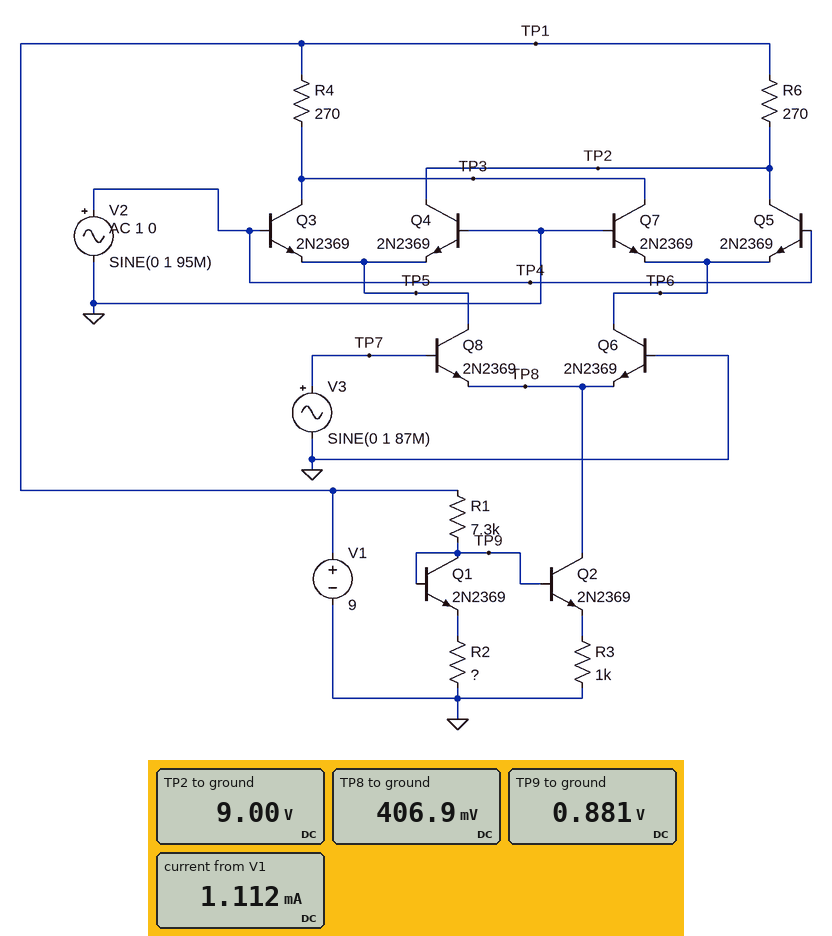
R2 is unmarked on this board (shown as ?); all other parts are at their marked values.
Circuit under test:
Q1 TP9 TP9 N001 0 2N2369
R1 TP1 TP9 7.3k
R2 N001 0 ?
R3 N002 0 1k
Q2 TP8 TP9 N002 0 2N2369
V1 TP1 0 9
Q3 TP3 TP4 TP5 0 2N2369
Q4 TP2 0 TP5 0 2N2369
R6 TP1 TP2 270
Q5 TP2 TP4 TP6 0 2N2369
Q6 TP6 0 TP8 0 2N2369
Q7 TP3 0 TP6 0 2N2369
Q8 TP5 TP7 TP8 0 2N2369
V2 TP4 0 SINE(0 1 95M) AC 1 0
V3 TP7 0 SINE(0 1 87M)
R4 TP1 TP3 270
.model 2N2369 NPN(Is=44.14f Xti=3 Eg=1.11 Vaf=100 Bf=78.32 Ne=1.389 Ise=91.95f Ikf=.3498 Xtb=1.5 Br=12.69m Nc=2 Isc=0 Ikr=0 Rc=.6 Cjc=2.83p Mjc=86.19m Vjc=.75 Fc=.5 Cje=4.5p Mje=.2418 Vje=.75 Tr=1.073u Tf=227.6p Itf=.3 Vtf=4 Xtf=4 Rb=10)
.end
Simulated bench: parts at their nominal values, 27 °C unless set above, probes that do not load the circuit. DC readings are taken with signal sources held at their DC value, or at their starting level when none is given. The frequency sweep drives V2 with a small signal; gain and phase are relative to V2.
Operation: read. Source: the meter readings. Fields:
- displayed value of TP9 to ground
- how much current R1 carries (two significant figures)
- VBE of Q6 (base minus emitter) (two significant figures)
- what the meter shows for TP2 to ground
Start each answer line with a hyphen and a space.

- 0.881 V
- 1.1 mA
- -410 mV
- 9.00 V
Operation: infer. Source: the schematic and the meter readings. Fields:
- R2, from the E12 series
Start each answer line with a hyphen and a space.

- 330 Ω
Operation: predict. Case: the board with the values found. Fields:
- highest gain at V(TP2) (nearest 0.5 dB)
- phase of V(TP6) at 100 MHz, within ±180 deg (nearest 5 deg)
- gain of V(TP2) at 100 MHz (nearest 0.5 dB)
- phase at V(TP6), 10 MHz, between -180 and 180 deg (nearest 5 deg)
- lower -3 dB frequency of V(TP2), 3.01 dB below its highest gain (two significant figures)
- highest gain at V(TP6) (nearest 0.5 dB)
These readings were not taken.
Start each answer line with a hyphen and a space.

- -6.5 dB
- 0 deg
- -10.5 dB
- 0 deg
- 120 MHz
- -8.5 dB
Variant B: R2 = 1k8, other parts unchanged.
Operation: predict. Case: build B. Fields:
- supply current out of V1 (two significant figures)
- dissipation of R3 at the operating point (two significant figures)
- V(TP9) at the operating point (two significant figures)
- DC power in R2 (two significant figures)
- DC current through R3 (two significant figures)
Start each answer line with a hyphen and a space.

- 1.1 mA
- 450 µW
- 1.3 V
- 270 µW
- 670 µA
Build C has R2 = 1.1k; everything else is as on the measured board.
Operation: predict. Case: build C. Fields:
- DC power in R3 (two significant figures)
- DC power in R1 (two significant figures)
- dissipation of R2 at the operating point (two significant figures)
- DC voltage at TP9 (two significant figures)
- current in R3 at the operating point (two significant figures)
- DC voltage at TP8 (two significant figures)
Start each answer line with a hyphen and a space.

- 310 µW
- 8.4 mW
- 290 µW
- 1.2 V
- 560 µA
- 670 mV
